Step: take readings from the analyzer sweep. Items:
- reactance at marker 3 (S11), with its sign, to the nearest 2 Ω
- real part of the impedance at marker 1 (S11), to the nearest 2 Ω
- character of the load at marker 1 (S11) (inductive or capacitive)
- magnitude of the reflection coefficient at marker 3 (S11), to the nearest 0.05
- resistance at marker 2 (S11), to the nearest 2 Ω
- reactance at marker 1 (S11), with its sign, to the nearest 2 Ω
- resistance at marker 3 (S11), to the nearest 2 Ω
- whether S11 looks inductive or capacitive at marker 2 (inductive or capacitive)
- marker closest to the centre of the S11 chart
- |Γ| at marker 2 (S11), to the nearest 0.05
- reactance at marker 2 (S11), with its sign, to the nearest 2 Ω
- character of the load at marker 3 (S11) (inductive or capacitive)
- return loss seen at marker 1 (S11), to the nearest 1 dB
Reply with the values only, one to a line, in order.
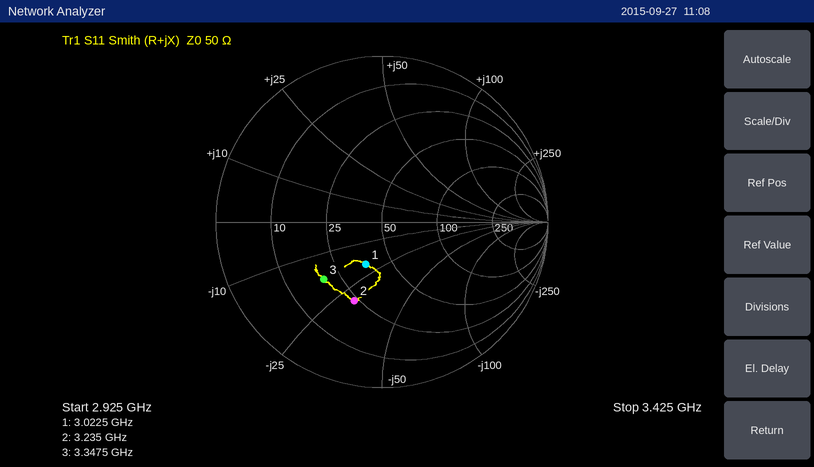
-18 Ω
36 Ω
capacitive
0.50
24 Ω
-20 Ω
20 Ω
capacitive
marker 1
0.50
-30 Ω
capacitive
11 dB
